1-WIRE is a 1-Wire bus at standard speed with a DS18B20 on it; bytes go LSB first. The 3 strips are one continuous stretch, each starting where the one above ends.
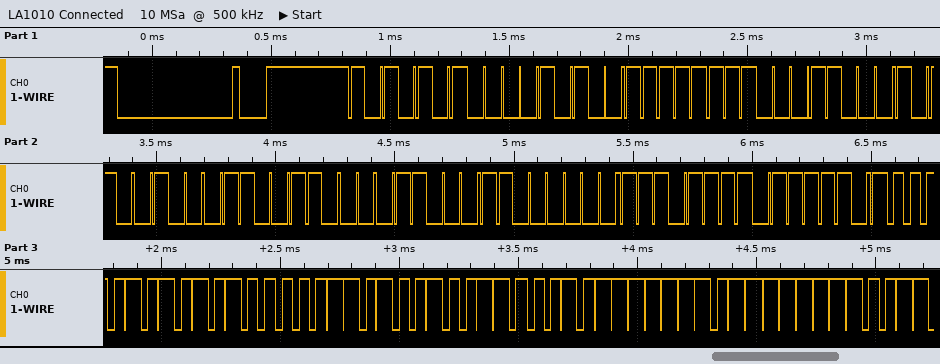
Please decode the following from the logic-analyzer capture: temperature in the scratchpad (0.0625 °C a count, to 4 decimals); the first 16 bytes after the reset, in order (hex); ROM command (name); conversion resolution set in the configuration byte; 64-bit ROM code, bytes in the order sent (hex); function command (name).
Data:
85.0000 °C
55 28 FF 18 25 66 18 03 F7 BE 50 05 4B 46 7F FF
Match ROM
12 bits
28 FF 18 25 66 18 03 F7
Read Scratchpad
